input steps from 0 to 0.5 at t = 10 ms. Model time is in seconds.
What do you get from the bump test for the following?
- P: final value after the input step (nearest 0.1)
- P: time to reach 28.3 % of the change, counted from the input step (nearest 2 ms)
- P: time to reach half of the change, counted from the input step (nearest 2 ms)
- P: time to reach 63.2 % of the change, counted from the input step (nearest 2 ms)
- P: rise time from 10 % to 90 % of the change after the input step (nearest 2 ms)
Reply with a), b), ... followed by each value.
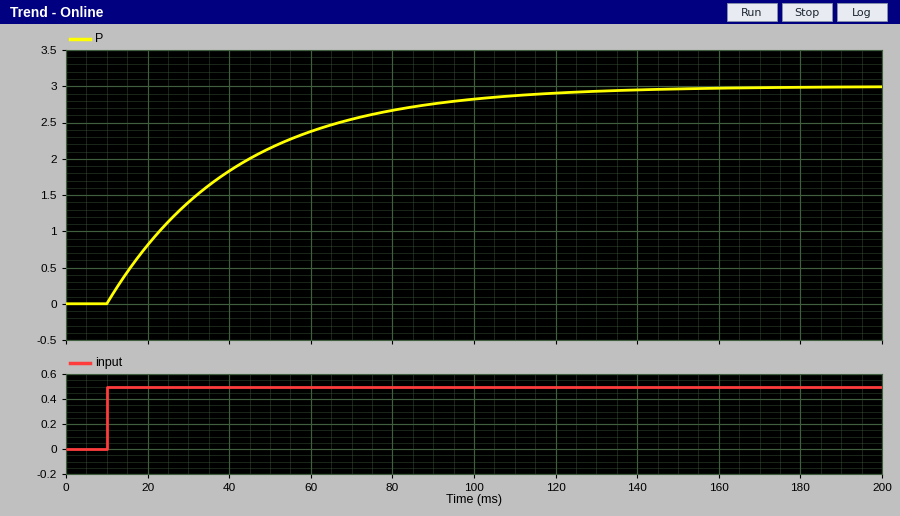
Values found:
a) 3.0
b) 10 ms
c) 22 ms
d) 32 ms
e) 70 ms
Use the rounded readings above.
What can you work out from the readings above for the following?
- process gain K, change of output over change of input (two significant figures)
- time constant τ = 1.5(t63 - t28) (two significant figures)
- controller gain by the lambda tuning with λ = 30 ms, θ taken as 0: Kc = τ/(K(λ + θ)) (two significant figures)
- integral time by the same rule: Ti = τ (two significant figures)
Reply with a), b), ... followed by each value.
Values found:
a) 6.0
b) 33 ms
c) 0.18
d) 33 ms
